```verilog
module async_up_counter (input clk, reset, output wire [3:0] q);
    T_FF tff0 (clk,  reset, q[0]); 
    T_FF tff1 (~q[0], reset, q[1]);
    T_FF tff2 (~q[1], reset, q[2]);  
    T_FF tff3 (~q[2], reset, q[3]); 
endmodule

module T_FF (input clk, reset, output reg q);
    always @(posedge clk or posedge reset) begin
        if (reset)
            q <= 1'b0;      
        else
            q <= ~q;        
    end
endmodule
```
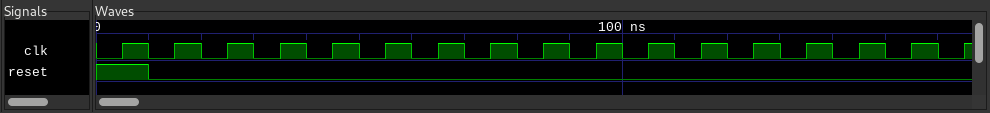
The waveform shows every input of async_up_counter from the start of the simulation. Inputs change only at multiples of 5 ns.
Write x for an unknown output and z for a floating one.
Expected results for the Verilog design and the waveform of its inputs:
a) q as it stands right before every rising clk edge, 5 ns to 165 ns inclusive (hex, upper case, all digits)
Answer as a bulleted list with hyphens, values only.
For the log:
- 0, 0, 1, 2, 3, 4, 5, 6, 7, 8, 9, A, B, C, D, E, F
